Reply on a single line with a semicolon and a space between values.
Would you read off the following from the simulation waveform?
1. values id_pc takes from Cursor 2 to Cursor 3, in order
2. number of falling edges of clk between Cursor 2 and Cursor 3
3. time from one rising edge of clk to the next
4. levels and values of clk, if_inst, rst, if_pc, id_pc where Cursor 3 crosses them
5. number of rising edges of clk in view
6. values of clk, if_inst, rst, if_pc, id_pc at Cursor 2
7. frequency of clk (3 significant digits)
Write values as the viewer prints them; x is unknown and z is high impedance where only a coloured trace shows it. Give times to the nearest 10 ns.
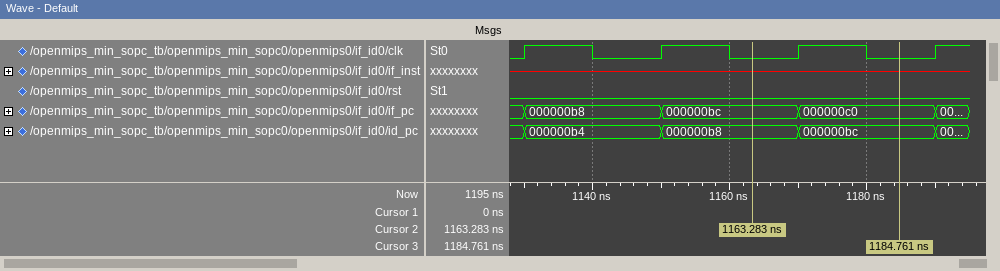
000000b8, 000000bc; 1; 20 ns; clk=0, if_inst=x, rst=0, if_pc=000000c0, id_pc=000000bc; 4; clk=0, if_inst=x, rst=0, if_pc=000000bc, id_pc=000000b8; 50.0 MHz
